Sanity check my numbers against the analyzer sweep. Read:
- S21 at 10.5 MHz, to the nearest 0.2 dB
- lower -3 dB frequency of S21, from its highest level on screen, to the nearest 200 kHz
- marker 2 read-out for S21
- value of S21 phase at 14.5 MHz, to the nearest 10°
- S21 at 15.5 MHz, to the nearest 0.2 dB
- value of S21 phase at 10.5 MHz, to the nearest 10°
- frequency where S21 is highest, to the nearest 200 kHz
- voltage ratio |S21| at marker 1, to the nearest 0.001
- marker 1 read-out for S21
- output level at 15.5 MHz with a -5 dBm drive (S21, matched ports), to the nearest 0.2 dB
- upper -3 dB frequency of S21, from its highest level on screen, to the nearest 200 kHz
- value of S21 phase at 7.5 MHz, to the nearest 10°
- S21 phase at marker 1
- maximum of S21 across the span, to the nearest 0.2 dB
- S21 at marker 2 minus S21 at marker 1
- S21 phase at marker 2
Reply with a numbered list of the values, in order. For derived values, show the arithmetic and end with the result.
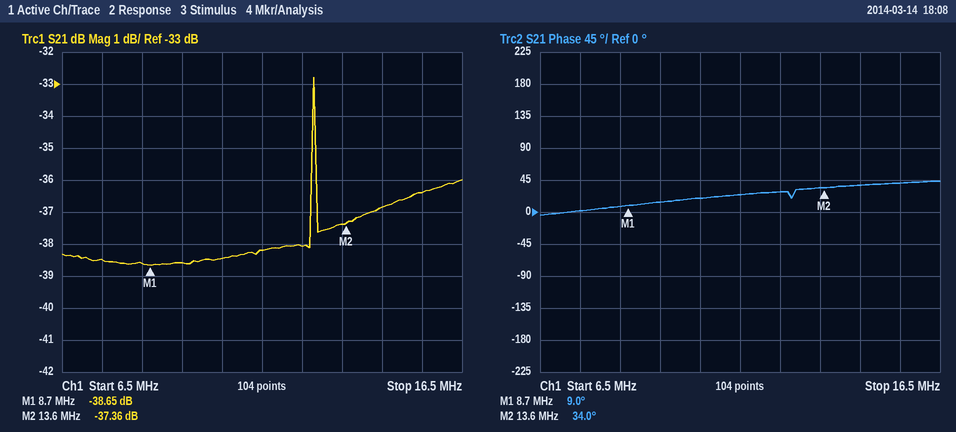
1. -38.4 dB
2. 12.8 MHz
3. -37.36 dB
4. 40°
5. -36.4 dB
6. 20°
7. 12.8 MHz
8. 10^(-38.65/20) ≈ 0.012
9. -38.65 dB
10. -5 dBm + (-36.4 dB) = -41.4 dBm
11. 12.8 MHz
12. 0°
13. 9.0°
14. -32.8 dB
15. -37.36 − (-38.65) = 1.29 dB
16. 34.0°
